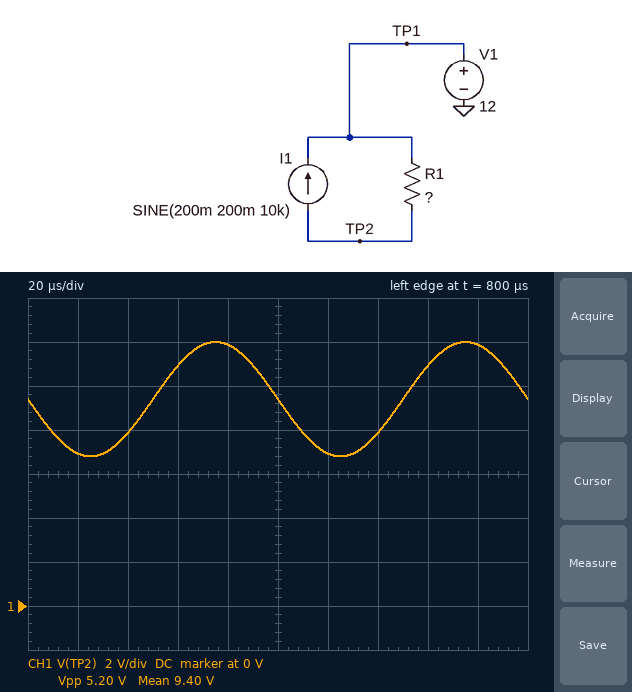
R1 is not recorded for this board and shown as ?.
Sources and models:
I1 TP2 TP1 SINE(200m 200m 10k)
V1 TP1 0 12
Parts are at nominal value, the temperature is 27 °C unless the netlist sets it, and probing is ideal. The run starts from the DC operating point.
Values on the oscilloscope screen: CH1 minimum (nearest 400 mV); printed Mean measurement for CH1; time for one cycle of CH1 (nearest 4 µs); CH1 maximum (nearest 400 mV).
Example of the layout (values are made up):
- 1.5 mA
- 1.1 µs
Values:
- 6.8 V
- 9.40 V
- 100 µs
- 12.0 V
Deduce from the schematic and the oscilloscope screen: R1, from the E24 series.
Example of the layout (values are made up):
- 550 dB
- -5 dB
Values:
- 13 Ω
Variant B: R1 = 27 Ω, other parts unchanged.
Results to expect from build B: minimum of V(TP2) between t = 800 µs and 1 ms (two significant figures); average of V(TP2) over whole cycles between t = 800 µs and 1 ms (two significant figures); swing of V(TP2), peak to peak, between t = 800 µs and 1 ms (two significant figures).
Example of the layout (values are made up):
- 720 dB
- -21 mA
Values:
- 1.2 V
- 6.6 V
- 11 V
